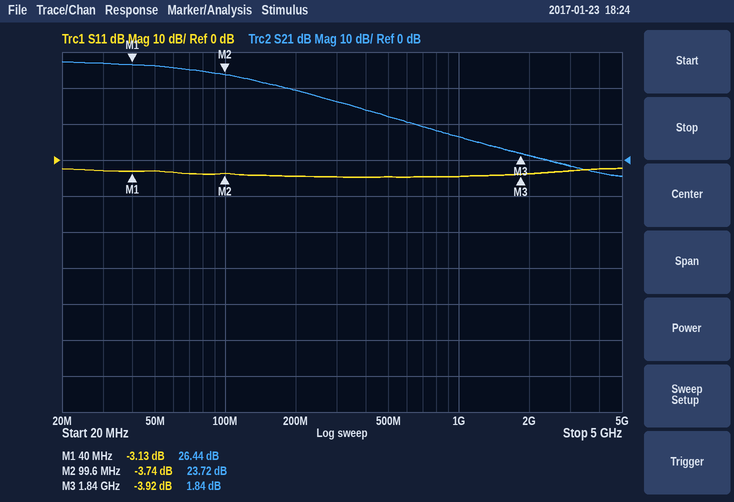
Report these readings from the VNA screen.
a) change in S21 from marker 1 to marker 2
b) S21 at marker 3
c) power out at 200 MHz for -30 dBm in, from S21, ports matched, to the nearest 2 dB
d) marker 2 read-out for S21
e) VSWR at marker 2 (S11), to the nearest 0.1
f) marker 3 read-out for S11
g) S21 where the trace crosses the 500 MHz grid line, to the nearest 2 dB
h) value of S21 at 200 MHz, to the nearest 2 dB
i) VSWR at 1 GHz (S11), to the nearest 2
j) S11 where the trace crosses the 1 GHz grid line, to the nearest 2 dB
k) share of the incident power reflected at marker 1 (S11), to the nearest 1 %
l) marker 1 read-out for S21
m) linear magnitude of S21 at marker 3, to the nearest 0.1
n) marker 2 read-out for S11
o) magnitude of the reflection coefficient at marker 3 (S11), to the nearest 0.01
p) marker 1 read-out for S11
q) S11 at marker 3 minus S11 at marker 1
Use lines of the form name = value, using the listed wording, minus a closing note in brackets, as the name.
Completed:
change in S21 from marker 1 to marker 2 = -2.72 dB
S21 at marker 3 = 1.84 dB
power out at 200 MHz for -30 dBm in, from S21, ports matched, to the nearest 2 dB = -10 dBm
marker 2 read-out for S21 = 23.72 dB
VSWR at marker 2 (S11), to the nearest 0.1 = 4.7
marker 3 read-out for S11 = -3.92 dB
S21 where the trace crosses the 500 MHz grid line, to the nearest 2 dB = 12 dB
value of S21 at 200 MHz, to the nearest 2 dB = 20 dB
VSWR at 1 GHz (S11), to the nearest 2 = 4
S11 where the trace crosses the 1 GHz grid line, to the nearest 2 dB = -4 dB
share of the incident power reflected at marker 1 (S11), to the nearest 1 % = 49 %
marker 1 read-out for S21 = 26.44 dB
linear magnitude of S21 at marker 3, to the nearest 0.1 = 1.2
marker 2 read-out for S11 = -3.74 dB
magnitude of the reflection coefficient at marker 3 (S11), to the nearest 0.01 = 0.64
marker 1 read-out for S11 = -3.13 dB
S11 at marker 3 minus S11 at marker 1 = -0.79 dB
